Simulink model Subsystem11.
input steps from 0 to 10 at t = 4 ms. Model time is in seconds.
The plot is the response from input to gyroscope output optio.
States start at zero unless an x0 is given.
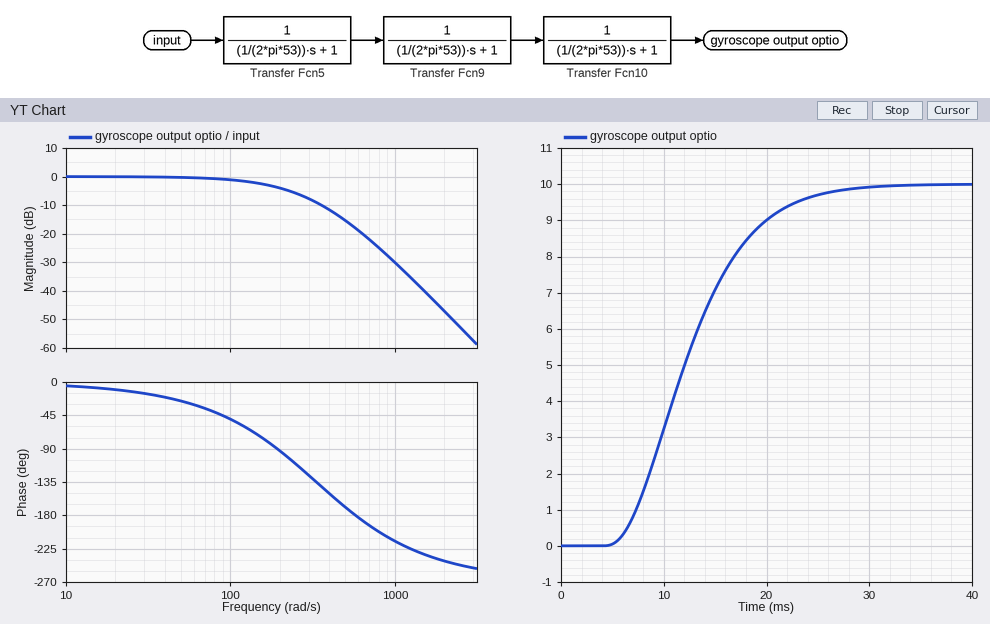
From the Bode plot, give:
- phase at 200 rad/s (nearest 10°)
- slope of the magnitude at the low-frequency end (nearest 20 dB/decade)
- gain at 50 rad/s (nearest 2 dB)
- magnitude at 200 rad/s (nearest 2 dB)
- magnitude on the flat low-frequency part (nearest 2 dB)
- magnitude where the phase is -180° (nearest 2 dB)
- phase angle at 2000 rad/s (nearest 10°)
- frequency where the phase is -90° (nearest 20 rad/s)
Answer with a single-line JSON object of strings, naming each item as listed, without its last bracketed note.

{"phase at 200 rad/s": "-90°", "slope of the magnitude at the low-frequency end": "0 dB/decade", "gain at 50 rad/s": "0 dB", "magnitude at 200 rad/s": "-4 dB", "magnitude on the flat low-frequency part": "0 dB", "magnitude where the phase is -180°": "-18 dB", "phase angle at 2000 rad/s": "-240°", "frequency where the phase is -90°": "200 rad/s"}
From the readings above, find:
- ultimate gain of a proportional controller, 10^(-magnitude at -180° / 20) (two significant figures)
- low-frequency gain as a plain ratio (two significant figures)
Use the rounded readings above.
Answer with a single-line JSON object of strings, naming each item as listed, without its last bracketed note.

{"ultimate gain of a proportional controller, 10^(-magnitude at -180° / 20)": "7.9", "low-frequency gain as a plain ratio": "1.0"}
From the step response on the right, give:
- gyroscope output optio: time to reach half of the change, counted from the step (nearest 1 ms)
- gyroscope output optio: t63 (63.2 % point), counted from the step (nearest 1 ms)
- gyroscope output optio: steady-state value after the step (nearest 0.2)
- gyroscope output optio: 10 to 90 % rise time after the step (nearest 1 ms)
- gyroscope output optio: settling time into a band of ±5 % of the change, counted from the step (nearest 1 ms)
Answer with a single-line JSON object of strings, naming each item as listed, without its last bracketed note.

{"gyroscope output optio: time to reach half of the change, counted from the step": "8 ms", "gyroscope output optio: t63 (63.2 % point), counted from the step": "10 ms", "gyroscope output optio: steady-state value after the step": "10.0", "gyroscope output optio: 10 to 90 % rise time after the step": "13 ms", "gyroscope output optio: settling time into a band of ±5 % of the change, counted from the step": "19 ms"}
